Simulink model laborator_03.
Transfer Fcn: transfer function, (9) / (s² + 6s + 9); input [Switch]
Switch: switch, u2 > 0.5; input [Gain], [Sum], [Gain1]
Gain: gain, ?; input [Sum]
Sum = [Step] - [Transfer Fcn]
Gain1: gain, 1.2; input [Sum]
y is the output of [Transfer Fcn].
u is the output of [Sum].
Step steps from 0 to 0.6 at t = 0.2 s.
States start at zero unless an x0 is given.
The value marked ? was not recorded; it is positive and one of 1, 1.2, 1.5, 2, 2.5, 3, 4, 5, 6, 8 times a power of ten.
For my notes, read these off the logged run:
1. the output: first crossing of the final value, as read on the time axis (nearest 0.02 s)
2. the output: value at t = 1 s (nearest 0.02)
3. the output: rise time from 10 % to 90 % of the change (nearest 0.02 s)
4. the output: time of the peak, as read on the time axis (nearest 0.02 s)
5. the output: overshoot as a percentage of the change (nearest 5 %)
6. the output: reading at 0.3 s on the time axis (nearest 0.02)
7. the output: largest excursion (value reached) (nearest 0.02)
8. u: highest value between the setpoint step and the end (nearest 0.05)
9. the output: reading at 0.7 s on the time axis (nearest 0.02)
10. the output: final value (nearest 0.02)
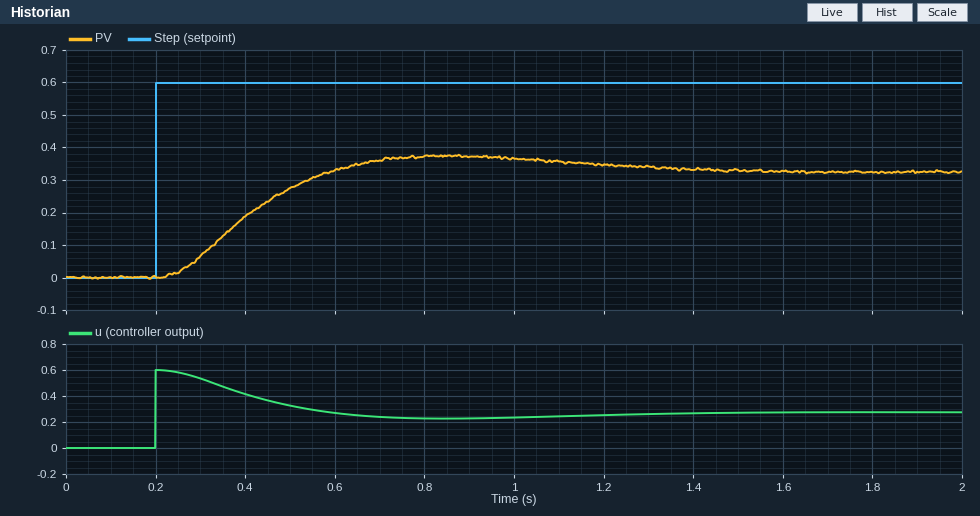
0.60 s
0.36
0.26 s
0.84 s
15 %
0.06
0.38
0.60
0.36
0.32
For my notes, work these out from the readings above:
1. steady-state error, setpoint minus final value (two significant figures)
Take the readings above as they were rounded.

0.28
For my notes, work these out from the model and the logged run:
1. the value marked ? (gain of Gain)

3
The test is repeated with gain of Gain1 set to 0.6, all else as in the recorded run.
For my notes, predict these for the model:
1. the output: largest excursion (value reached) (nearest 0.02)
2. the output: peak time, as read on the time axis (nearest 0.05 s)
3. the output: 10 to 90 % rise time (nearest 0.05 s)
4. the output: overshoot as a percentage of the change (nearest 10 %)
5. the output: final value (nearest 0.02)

0.30
0.75 s
0.15 s
30 %
0.22
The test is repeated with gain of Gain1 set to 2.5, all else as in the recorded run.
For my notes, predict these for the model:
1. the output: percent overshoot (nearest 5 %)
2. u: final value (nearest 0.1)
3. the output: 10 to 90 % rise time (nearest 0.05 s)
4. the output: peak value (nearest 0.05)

15 %
0.2
0.30 s
0.50
